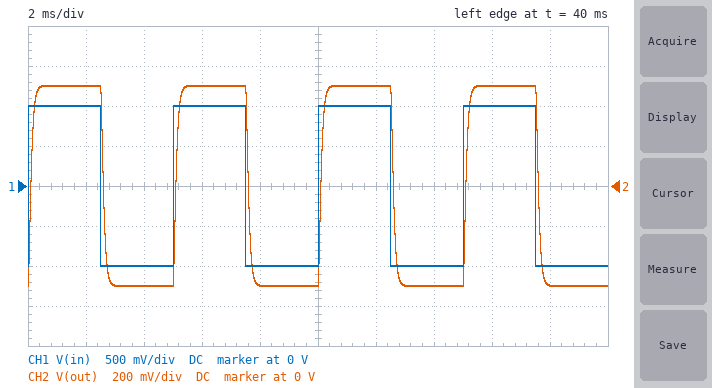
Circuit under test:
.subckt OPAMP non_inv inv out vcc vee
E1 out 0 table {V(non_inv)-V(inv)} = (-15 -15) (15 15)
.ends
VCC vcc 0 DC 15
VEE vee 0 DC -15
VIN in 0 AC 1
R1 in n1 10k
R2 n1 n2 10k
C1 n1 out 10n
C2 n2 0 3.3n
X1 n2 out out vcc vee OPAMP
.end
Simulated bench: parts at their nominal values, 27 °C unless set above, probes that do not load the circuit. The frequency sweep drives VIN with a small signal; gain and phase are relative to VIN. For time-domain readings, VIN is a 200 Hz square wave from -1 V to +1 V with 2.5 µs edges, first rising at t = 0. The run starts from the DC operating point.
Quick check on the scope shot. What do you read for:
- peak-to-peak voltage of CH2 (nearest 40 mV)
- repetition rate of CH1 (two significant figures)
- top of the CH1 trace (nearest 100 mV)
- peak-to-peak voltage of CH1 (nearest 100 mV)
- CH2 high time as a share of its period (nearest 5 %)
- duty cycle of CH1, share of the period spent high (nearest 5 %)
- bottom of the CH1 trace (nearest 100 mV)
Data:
1.00 V
200 Hz
1.0 V
2.0 V
50 %
50 %
-1.0 V
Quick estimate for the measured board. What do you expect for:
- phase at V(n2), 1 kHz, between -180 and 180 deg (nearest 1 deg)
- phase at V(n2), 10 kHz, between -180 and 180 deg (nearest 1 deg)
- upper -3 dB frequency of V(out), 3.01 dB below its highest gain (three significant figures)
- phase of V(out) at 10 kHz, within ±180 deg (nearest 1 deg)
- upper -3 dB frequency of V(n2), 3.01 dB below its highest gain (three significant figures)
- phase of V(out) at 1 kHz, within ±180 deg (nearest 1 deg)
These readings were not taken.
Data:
-40 deg
-149 deg
1.76 kHz
-149 deg
1.76 kHz
-40 deg
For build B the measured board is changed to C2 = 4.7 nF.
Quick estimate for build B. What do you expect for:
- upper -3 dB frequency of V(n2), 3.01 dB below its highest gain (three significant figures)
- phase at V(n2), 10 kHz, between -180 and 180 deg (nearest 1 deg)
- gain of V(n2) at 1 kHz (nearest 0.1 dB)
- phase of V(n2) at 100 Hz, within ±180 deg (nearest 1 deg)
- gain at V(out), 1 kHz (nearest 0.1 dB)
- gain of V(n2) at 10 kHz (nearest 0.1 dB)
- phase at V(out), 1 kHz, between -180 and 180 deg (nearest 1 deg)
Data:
1.39 kHz
-153 deg
-1.7 dB
-5 deg
-7.7 dB
-25.9 dB
-48 deg
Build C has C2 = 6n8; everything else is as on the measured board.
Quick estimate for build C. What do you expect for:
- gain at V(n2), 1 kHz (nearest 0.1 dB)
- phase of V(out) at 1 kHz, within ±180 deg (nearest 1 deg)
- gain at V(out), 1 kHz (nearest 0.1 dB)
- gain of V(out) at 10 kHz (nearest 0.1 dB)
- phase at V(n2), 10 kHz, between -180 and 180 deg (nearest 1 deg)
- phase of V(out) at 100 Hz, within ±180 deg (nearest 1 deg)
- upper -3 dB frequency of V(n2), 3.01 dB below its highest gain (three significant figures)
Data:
-2.8 dB
-58 deg
-8.8 dB
-35.1 dB
-156 deg
-7 deg
1.05 kHz
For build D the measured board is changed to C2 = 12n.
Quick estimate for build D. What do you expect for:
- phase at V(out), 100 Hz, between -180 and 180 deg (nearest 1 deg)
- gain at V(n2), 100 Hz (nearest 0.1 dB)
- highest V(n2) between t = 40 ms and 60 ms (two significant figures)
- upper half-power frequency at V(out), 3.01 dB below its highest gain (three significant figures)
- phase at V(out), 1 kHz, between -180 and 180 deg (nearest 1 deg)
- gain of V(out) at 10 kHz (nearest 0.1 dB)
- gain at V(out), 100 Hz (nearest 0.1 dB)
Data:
-10 deg
-0.1 dB
1.0 V
637 Hz
-74 deg
-40.0 dB
-6.1 dB
